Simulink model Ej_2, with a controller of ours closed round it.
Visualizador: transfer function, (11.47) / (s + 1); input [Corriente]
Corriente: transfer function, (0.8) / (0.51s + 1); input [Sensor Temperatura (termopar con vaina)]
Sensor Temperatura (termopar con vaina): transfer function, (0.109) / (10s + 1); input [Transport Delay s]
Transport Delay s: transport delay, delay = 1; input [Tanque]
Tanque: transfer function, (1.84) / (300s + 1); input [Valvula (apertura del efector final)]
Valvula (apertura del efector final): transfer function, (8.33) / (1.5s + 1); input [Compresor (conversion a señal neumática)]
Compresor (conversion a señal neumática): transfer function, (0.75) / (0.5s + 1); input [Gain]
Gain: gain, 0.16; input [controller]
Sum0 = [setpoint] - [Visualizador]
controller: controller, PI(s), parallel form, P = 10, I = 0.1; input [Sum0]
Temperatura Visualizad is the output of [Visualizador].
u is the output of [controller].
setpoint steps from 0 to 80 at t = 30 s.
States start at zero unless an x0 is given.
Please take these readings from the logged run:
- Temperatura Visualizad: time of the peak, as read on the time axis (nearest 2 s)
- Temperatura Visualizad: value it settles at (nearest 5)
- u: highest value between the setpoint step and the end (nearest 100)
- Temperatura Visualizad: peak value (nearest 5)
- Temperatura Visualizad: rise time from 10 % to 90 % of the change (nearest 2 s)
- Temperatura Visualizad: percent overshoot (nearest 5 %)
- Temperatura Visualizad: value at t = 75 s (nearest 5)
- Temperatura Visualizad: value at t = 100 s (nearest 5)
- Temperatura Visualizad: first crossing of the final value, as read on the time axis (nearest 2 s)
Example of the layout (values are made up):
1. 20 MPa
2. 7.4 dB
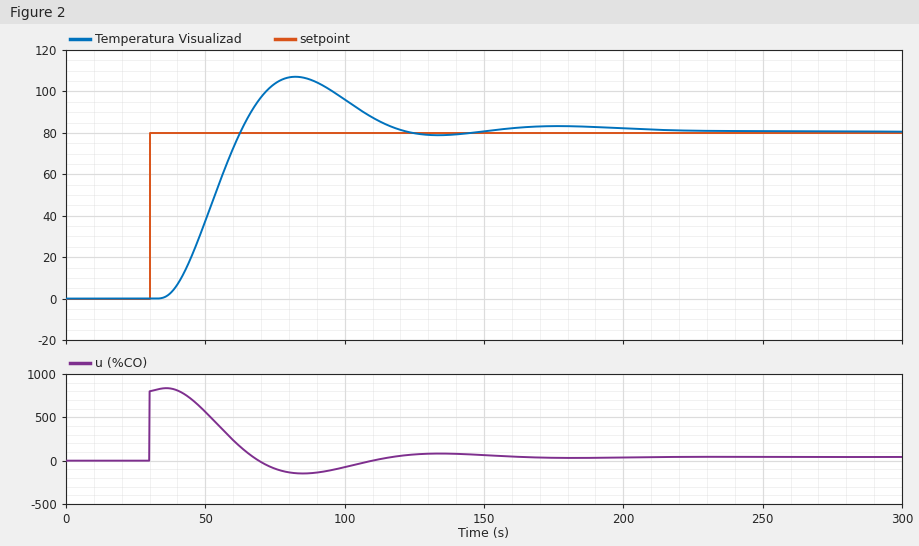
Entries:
1. 82 s
2. 80
3. 800
4. 105
5. 20 s
6. 35 %
7. 105
8. 95
9. 62 s
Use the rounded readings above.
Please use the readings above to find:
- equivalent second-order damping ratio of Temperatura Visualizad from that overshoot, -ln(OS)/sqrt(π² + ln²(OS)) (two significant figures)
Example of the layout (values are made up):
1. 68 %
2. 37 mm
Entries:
1. 0.32
